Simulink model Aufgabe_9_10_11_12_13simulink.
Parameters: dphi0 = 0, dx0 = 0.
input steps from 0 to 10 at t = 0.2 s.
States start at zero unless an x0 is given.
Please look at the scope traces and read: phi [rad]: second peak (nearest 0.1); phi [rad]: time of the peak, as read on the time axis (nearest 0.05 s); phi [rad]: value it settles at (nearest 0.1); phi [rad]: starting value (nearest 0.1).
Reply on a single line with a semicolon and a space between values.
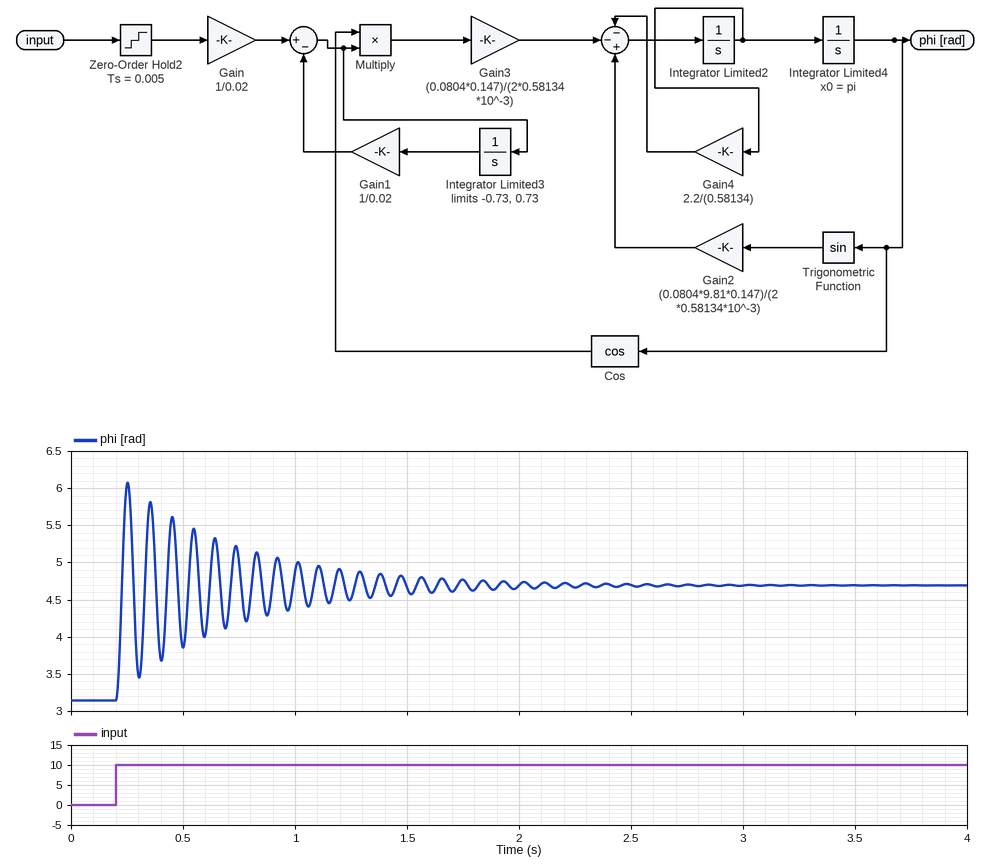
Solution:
5.8; 0.25 s; 4.7; 3.1
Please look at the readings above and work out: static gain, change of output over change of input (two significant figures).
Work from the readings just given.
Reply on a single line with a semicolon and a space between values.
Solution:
0.16
